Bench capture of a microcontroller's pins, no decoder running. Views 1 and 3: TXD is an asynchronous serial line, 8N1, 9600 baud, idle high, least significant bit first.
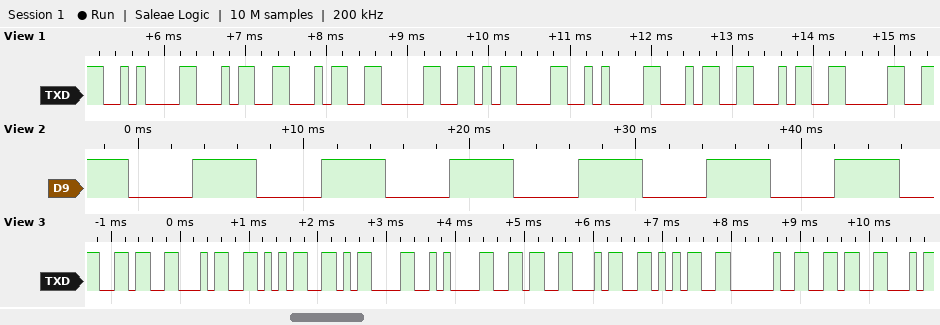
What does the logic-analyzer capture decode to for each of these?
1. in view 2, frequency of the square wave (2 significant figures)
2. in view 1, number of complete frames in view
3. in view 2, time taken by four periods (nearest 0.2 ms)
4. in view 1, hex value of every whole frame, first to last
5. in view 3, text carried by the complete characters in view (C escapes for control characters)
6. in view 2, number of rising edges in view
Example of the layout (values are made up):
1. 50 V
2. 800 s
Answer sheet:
1. 130 Hz
2. 9
3. 31.0 ms
4. 0A 34 34 30 0D 0A 34 34 30
5. "645\r\n645 6"
6. 6
